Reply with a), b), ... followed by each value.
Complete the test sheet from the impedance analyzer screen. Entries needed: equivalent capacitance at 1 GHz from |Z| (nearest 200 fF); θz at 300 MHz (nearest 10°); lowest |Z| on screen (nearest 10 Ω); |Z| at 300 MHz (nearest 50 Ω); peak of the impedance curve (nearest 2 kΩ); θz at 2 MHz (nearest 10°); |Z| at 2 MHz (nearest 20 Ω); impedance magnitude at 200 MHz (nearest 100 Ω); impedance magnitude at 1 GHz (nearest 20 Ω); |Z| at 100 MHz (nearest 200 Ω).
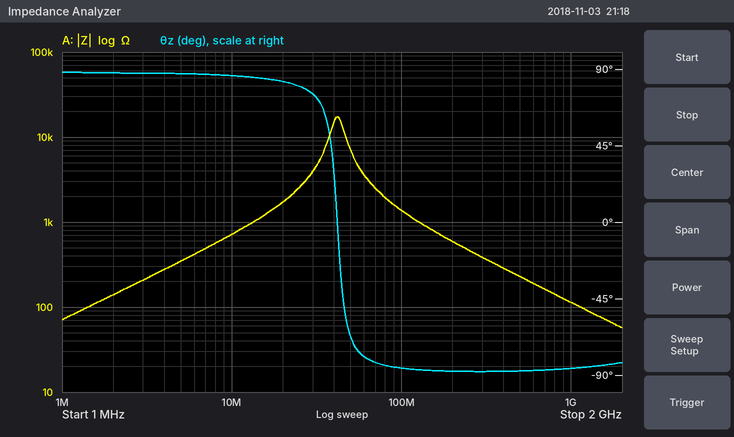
a) 1.4 pF
b) -90°
c) 60 Ω
d) 400 Ω
e) 18 kΩ
f) 90°
g) 140 Ω
h) 600 Ω
i) 120 Ω
j) 1.4 kΩ
